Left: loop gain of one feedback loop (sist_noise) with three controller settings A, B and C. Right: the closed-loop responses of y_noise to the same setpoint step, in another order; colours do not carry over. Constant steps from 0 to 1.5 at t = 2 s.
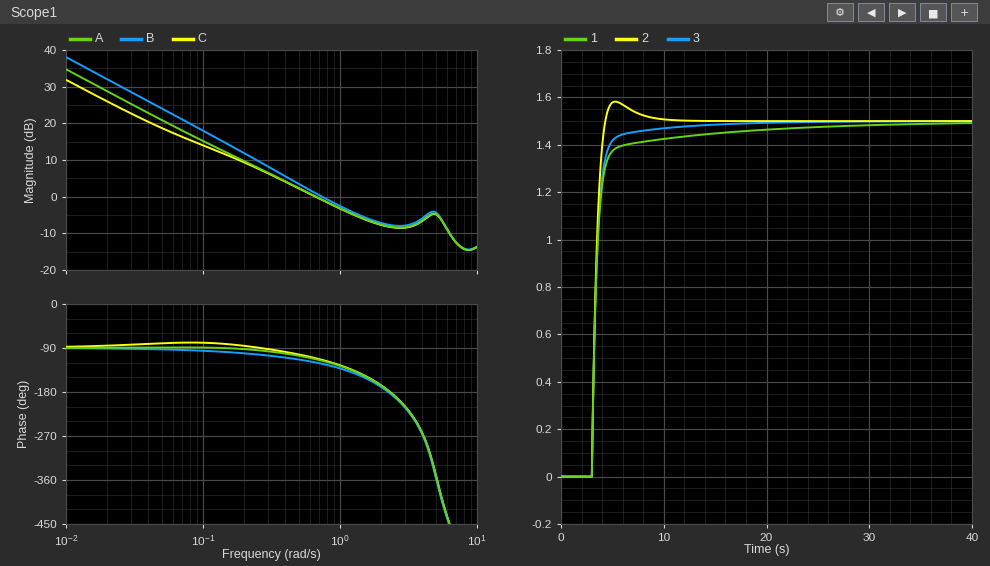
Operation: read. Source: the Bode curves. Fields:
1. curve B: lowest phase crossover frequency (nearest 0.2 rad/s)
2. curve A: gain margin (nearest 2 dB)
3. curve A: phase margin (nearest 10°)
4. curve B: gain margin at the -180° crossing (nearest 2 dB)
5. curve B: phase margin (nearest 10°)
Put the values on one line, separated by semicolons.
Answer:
2.2 rad/s; 8 dB; 70°; 8 dB; 60°
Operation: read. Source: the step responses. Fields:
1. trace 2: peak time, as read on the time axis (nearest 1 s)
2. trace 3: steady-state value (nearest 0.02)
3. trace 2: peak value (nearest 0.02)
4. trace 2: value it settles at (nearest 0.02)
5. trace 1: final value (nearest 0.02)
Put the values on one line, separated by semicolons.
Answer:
5 s; 1.50; 1.58; 1.50; 1.50
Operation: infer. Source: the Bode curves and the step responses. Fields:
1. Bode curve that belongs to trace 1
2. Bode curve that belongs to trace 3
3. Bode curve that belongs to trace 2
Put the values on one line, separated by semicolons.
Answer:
C; A; B
